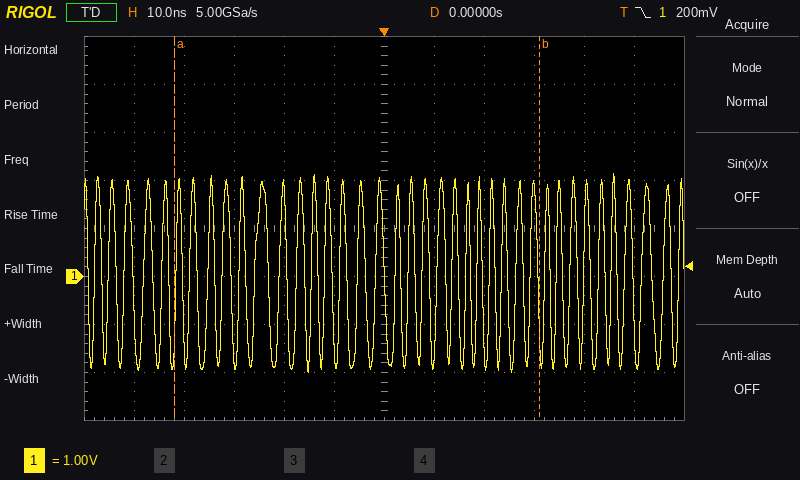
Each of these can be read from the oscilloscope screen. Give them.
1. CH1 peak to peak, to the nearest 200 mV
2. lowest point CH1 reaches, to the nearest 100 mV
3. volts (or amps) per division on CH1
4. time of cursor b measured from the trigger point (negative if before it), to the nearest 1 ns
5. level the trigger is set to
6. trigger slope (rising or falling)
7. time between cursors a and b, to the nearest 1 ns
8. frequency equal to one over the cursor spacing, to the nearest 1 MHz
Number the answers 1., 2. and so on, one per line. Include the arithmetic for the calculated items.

1. 4.2 V
2. -2.0 V
3. 1 V
4. +31 ns
5. 200 mV
6. falling
7. 73 ns
8. 1 / 73 ns ≈ 14 MHz
